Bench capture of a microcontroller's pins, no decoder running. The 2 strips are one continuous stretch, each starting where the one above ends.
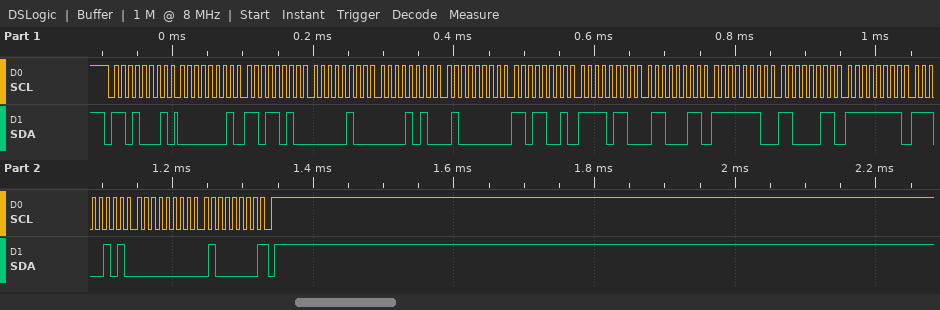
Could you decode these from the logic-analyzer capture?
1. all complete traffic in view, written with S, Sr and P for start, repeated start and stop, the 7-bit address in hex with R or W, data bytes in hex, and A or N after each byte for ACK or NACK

S 68R A 01 A DA A 04 A 0A A 40 A D9 A F6 A 63 A FE A C3 A FF A E5 A 00 A 40 N P
